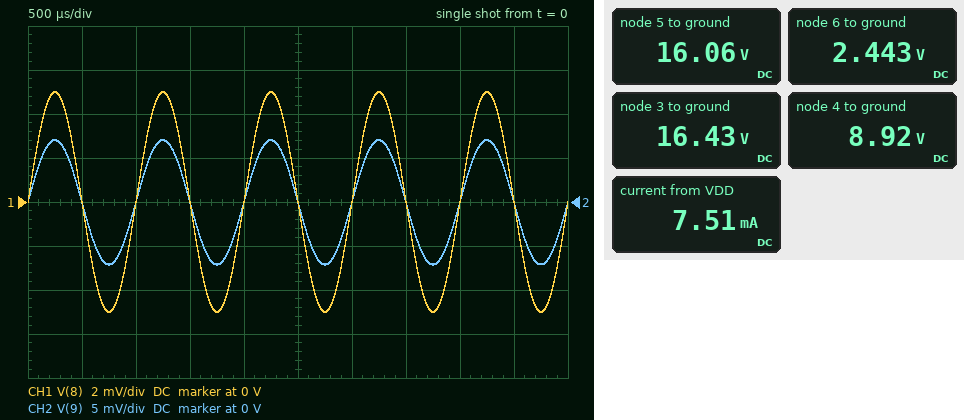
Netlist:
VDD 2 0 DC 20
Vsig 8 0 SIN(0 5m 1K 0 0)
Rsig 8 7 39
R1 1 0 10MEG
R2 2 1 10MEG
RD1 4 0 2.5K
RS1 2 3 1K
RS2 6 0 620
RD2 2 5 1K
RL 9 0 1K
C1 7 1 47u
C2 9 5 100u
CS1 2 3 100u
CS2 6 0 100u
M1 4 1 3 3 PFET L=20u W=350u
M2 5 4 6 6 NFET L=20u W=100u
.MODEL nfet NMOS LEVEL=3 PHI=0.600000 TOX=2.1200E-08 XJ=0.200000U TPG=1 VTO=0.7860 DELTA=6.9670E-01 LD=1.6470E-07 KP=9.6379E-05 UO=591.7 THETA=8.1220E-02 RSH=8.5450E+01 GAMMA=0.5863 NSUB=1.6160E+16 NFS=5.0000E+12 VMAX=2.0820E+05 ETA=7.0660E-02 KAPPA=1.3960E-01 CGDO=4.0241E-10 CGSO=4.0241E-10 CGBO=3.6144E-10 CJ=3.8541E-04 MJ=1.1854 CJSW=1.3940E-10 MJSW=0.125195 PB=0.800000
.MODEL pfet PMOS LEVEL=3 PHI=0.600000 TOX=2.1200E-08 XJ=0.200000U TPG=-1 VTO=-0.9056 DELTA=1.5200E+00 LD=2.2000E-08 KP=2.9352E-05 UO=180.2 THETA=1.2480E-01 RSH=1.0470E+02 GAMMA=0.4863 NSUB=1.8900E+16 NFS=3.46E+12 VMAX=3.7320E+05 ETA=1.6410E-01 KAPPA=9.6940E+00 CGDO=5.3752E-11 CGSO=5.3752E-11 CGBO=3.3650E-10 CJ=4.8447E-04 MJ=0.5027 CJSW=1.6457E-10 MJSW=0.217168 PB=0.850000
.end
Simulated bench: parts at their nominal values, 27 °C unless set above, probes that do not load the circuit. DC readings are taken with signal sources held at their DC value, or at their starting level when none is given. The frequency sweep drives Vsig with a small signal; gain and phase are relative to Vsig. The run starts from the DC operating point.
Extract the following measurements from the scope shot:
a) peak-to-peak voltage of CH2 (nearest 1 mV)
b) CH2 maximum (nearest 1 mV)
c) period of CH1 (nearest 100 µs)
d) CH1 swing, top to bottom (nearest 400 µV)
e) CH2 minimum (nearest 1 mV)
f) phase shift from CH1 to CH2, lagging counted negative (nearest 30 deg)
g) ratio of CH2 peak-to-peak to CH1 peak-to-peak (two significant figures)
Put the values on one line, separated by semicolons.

14 mV; 7 mV; 1.0 ms; 10.0 mV; -7 mV; 0 deg; 1.4
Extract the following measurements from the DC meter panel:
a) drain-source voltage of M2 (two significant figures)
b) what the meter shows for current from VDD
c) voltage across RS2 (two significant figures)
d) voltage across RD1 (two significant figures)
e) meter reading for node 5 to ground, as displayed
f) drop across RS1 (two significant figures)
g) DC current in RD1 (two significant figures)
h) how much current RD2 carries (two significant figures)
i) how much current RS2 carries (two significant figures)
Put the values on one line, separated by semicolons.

14 V; 7.51 mA; 2.4 V; 8.9 V; 16.06 V; 3.6 V; 3.6 mA; 3.9 mA; 3.9 mA
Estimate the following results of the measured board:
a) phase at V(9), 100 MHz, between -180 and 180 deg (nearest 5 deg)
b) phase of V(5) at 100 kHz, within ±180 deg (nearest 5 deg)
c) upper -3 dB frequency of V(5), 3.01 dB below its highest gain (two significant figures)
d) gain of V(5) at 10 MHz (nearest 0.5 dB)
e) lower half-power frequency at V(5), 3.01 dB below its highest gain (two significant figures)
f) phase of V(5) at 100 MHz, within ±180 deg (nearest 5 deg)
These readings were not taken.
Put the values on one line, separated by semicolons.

-110 deg; 0 deg; 29 MHz; 2.5 dB; 3.9 Hz; -110 deg
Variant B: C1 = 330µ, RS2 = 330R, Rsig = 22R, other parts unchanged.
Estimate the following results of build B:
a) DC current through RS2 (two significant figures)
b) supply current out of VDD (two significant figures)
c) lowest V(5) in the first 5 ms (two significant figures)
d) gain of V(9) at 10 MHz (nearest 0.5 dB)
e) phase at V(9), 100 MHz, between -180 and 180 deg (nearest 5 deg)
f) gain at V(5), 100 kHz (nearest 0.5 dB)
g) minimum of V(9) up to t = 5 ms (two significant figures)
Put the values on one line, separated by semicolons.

4.9 mA; 8.5 mA; 15 V; 3.0 dB; -105 deg; 3.5 dB; -7.6 mV
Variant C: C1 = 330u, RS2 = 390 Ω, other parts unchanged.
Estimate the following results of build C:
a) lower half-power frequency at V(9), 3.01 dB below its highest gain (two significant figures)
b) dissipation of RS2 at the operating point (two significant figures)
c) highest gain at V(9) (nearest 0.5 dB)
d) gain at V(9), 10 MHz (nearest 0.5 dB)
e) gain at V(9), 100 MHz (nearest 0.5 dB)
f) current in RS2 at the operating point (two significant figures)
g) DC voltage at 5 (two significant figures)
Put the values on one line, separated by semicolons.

4.7 Hz; 8.5 mW; 3.5 dB; 3.0 dB; -8.5 dB; 4.7 mA; 15 V
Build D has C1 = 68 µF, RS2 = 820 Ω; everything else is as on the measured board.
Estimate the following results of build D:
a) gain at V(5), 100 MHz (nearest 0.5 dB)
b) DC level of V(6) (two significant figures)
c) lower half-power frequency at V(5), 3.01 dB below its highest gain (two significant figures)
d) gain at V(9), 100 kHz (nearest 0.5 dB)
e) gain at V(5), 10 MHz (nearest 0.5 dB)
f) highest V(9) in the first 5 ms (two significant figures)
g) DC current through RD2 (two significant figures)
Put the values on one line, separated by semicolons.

-9.5 dB; 2.9 V; 3.7 Hz; 2.5 dB; 2.0 dB; 6.8 mV; 3.5 mA
